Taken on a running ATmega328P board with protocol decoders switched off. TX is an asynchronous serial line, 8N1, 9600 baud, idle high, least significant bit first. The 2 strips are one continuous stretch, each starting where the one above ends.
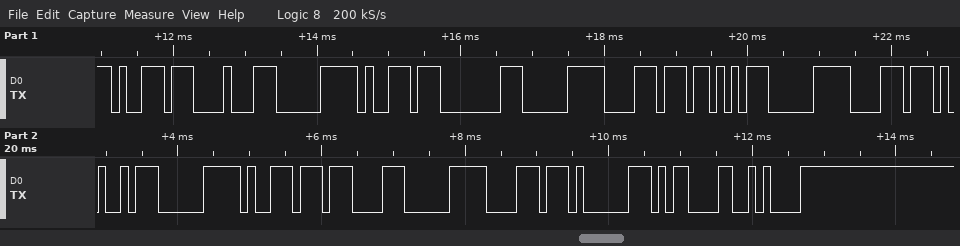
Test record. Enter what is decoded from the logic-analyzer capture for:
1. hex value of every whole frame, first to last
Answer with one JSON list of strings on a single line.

["B9 88 E0 B9 80 E0 B8 AB E0 B8 A5 E0 B9 87 E0 B8 81 0D 0A"]
